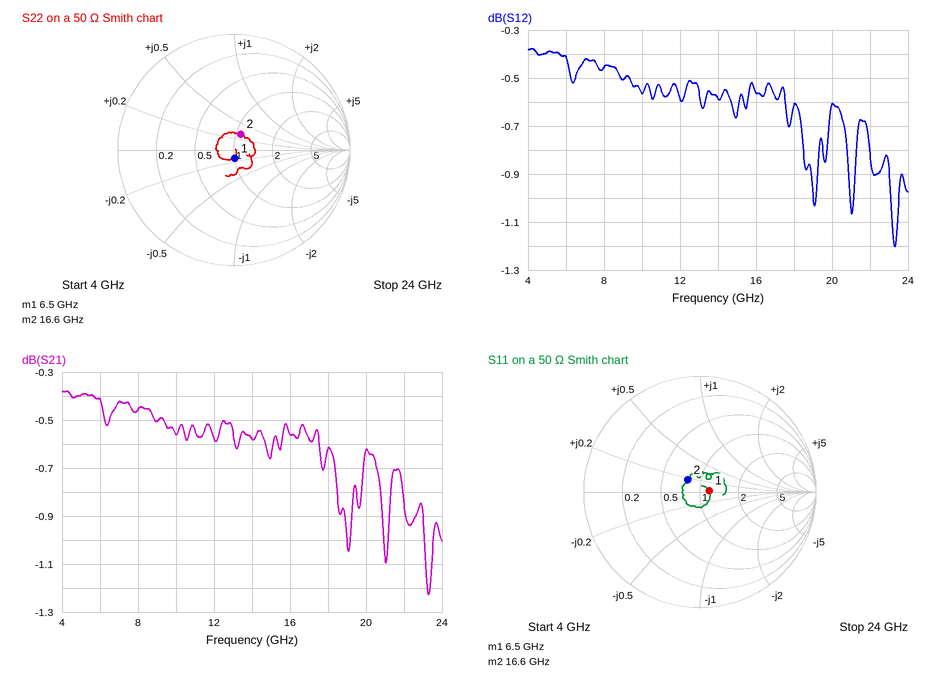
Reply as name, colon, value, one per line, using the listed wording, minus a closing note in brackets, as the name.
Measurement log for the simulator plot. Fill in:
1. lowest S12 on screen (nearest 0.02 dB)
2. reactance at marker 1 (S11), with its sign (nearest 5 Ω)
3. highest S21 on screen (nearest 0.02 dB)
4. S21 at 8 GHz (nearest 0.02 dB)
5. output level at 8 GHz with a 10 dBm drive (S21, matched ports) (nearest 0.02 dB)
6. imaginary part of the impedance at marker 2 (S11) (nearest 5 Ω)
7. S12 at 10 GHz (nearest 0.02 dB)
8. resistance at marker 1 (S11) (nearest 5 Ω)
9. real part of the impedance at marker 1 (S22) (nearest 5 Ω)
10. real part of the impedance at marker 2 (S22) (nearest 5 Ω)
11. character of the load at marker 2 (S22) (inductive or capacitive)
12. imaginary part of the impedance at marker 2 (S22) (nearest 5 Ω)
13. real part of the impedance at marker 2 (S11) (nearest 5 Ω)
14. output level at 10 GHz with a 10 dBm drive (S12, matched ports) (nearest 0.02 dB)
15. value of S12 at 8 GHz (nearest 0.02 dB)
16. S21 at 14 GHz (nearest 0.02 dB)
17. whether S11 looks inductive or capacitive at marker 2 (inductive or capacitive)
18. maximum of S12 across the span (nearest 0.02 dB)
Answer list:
lowest S12 on screen: -1.20 dB
reactance at marker 1 (S11), with its sign: 0 Ω
highest S21 on screen: -0.38 dB
S21 at 8 GHz: -0.46 dB
output level at 8 GHz with a 10 dBm drive (S21, matched ports): 9.54 dBm
imaginary part of the impedance at marker 2 (S11): +10 Ω
S12 at 10 GHz: -0.56 dB
resistance at marker 1 (S11): 60 Ω
real part of the impedance at marker 1 (S22): 50 Ω
real part of the impedance at marker 2 (S22): 55 Ω
character of the load at marker 2 (S22): inductive
imaginary part of the impedance at marker 2 (S22): +15 Ω
real part of the impedance at marker 2 (S11): 40 Ω
output level at 10 GHz with a 10 dBm drive (S12, matched ports): 9.44 dBm
value of S12 at 8 GHz: -0.46 dB
S21 at 14 GHz: -0.58 dB
whether S11 looks inductive or capacitive at marker 2: inductive
maximum of S12 across the span: -0.38 dB
